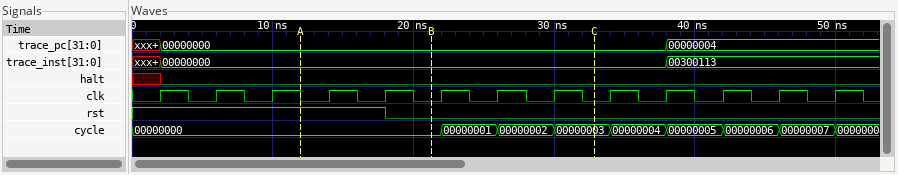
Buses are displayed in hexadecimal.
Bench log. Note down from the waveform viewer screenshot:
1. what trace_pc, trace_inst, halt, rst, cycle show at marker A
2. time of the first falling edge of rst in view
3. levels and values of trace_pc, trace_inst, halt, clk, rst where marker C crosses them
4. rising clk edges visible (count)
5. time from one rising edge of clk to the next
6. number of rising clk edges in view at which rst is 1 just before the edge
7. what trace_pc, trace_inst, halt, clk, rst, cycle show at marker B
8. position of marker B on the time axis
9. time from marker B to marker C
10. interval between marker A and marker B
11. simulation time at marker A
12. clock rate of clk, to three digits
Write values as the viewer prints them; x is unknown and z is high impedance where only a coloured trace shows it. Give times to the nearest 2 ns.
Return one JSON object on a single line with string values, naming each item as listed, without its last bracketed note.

{"what trace_pc, trace_inst, halt, rst, cycle show at marker A": "trace_pc=00000000, trace_inst=00000000, halt=0, rst=1, cycle=00000000", "time of the first falling edge of rst in view": "18 ns", "levels and values of trace_pc, trace_inst, halt, clk, rst where marker C crosses them": "trace_pc=00000000, trace_inst=00000000, halt=0, clk=0, rst=0", "rising clk edges visible": "13", "time from one rising edge of clk to the next": "4 ns", "number of rising clk edges in view at which rst is 1 just before the edge": "5", "what trace_pc, trace_inst, halt, clk, rst, cycle show at marker B": "trace_pc=00000000, trace_inst=00000000, halt=0, clk=0, rst=0, cycle=00000000", "position of marker B on the time axis": "22 ns", "time from marker B to marker C": "12 ns", "interval between marker A and marker B": "10 ns", "simulation time at marker A": "12 ns", "clock rate of clk, to three digits": "250 MHz"}
